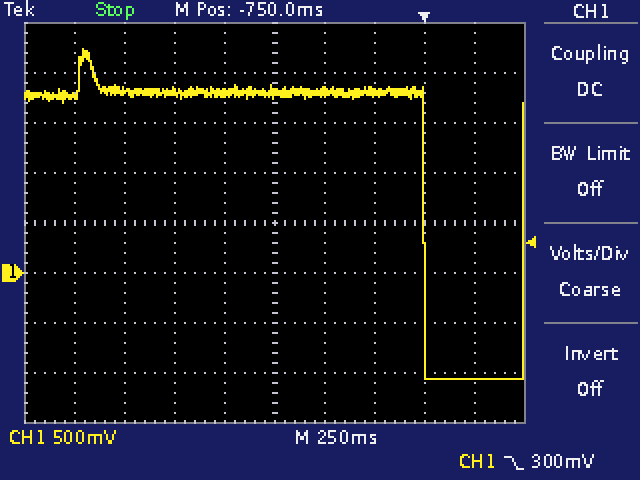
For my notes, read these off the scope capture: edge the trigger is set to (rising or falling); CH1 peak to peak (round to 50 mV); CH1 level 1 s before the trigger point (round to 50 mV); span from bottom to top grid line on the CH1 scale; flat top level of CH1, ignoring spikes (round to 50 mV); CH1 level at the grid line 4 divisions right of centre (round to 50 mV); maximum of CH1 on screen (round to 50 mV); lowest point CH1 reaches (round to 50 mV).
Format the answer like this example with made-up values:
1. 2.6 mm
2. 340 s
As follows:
1. falling
2. 3.30 V
3. 1.80 V
4. 4 V
5. 1.80 V
6. -1.05 V
7. 2.25 V
8. -1.05 V
